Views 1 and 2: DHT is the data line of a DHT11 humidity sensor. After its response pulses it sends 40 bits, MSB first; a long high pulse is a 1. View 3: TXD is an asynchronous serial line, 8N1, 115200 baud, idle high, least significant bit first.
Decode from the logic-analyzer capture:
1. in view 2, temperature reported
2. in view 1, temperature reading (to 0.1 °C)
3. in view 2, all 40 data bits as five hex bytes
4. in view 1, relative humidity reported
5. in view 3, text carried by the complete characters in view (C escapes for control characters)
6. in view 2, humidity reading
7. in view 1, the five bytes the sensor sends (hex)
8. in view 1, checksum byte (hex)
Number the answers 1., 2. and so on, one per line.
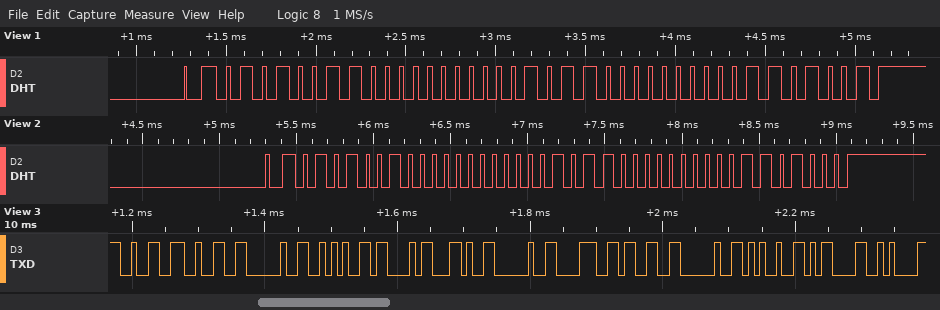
1. 22.0 °C
2. 22.0 °C
3. 52 00 16 00 68
4. 83 %
5. "22 *C, 83 %\r\n"
6. 82 %
7. 53 00 16 00 69
8. 0x69
